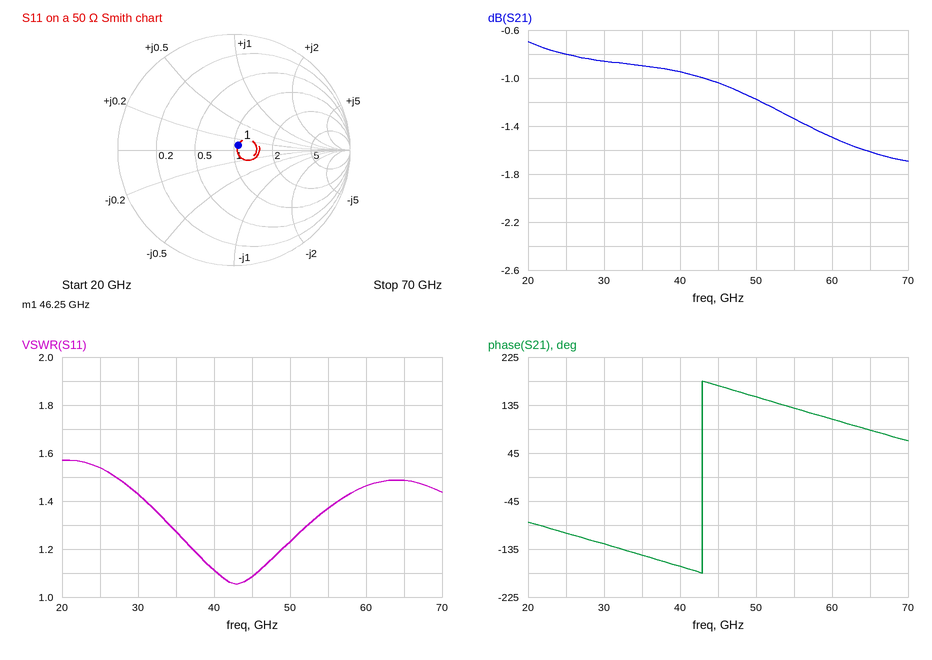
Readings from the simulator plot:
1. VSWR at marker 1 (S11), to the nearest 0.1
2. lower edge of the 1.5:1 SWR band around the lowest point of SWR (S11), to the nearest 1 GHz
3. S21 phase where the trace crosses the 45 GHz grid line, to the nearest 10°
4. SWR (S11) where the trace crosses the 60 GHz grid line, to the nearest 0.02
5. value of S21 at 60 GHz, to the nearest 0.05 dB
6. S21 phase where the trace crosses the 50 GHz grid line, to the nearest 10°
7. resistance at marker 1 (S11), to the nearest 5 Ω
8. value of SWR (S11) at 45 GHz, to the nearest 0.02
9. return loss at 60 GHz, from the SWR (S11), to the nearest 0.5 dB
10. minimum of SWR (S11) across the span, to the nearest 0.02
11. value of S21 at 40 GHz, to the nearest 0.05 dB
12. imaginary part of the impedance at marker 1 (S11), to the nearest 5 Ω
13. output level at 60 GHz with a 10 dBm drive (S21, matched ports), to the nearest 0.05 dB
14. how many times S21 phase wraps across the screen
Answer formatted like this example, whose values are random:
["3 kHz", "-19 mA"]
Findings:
["1.1", "27 GHz", "170°", "1.46", "-1.50 dB", "150°", "55 Ω", "1.08", "14.5 dB", "1.06", "-0.95 dB", "+5 Ω", "8.50 dBm", "1"]
